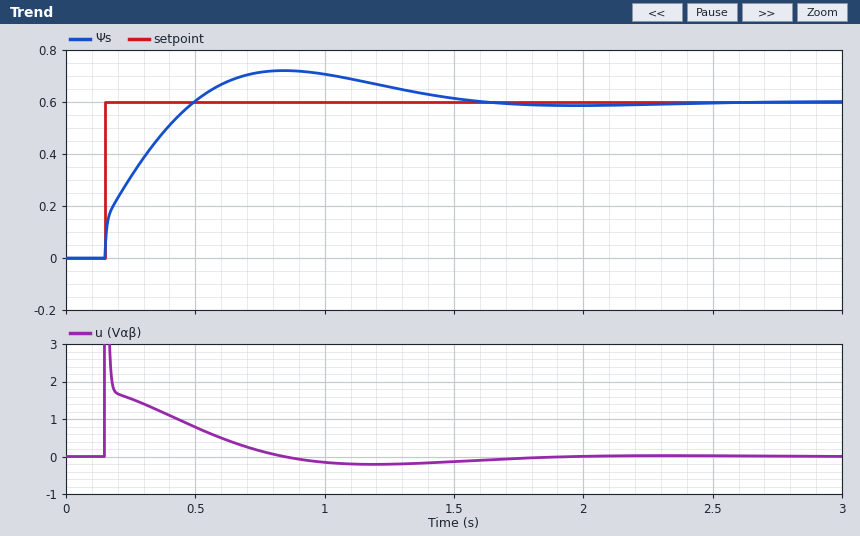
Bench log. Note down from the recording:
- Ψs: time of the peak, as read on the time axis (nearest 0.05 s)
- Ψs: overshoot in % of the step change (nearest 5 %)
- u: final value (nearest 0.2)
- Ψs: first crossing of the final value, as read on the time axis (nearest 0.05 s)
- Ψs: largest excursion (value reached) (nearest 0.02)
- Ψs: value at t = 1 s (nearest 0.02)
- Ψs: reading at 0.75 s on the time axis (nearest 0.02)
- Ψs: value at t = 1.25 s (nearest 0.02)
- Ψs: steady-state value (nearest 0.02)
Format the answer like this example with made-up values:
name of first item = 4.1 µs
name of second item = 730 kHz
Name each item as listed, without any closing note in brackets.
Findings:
Ψs: time of the peak, as read on the time axis = 0.85 s
Ψs: overshoot in % of the step change = 20 %
u: final value = 0.0
Ψs: first crossing of the final value, as read on the time axis = 0.50 s
Ψs: largest excursion (value reached) = 0.72
Ψs: value at t = 1 s = 0.70
Ψs: reading at 0.75 s on the time axis = 0.72
Ψs: value at t = 1.25 s = 0.66
Ψs: steady-state value = 0.60
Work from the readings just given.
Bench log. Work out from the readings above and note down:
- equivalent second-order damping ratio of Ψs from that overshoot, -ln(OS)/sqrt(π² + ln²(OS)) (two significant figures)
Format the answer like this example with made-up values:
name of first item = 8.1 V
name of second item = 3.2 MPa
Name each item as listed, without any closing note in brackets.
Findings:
equivalent second-order damping ratio of Ψs from that overshoot, -ln(OS)/sqrt(π² + ln²(OS)) = 0.46
